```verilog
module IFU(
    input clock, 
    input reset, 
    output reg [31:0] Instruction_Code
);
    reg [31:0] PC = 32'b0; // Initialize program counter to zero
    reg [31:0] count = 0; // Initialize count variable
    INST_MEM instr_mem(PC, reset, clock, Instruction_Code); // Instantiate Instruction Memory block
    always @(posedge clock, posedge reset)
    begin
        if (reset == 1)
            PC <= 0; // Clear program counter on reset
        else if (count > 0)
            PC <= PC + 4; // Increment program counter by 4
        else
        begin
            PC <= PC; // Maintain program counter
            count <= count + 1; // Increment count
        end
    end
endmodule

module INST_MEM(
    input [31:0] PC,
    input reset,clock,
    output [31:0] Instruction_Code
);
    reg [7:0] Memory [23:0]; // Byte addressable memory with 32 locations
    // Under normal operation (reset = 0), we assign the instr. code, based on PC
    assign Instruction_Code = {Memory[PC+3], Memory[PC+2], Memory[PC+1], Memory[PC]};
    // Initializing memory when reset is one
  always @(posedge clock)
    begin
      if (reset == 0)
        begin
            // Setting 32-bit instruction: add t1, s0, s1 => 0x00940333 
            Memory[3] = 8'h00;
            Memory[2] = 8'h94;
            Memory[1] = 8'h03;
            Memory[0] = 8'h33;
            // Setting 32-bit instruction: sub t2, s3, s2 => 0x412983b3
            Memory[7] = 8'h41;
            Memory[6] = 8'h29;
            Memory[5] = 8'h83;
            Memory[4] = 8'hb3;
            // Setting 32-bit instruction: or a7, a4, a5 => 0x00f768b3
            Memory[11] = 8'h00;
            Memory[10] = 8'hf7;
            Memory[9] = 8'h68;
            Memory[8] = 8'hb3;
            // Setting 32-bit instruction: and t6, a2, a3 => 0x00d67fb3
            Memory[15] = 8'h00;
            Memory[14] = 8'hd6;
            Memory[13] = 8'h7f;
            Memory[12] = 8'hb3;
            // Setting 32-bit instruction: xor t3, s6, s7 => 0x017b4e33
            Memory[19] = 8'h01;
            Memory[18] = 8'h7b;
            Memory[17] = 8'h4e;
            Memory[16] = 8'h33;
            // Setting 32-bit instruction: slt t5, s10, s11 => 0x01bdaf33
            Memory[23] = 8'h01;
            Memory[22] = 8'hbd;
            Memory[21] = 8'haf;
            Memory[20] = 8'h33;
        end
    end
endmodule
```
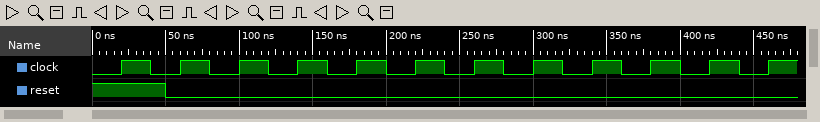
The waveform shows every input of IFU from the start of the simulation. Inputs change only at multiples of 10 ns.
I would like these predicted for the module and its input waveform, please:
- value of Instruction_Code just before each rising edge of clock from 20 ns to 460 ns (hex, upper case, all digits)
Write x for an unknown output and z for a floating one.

x, x, 00940333, 412983B3, 00F768B3, 00D67FB3, 017B4E33, 01BDAF33, x, x, x, x
